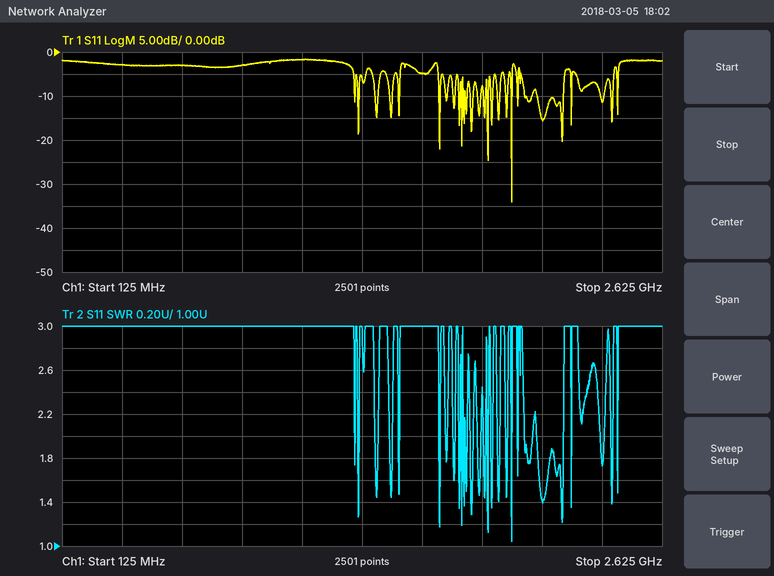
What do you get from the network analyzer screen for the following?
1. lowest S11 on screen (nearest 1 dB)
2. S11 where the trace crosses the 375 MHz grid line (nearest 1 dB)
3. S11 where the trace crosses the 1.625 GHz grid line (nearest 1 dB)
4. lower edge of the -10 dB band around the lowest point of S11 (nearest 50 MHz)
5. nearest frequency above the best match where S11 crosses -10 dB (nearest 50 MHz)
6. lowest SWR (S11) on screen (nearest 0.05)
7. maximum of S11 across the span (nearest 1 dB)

-34 dB
-3 dB
-5 dB
2.00 GHz
2.00 GHz
1.05
-2 dB
